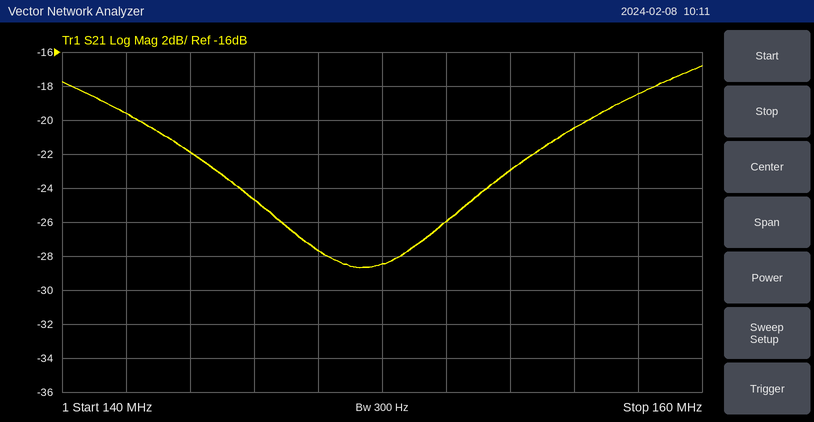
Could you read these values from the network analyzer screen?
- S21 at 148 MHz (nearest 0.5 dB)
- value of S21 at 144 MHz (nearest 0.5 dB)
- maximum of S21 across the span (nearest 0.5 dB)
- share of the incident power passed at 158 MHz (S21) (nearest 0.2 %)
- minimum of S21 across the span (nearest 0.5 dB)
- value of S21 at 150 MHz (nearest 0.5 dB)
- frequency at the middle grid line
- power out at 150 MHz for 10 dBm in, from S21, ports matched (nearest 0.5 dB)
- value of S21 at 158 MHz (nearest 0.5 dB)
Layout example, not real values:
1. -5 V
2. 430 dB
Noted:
1. -27.5 dB
2. -22.0 dB
3. -17.0 dB
4. 1.4 %
5. -28.5 dB
6. -28.5 dB
7. 150 MHz
8. -18.5 dBm
9. -18.5 dB
